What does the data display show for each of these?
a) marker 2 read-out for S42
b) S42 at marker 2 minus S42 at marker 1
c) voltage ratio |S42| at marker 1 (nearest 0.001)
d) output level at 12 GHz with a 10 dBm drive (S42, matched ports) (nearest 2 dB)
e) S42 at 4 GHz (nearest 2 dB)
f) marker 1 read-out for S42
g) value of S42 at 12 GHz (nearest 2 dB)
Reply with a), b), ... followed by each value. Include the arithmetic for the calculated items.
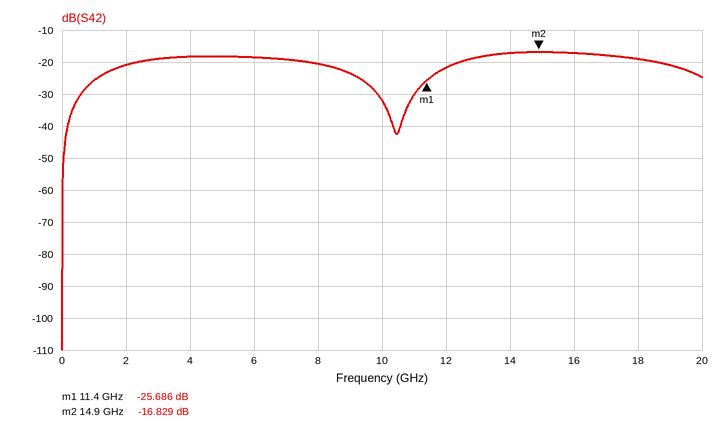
a) -16.829 dB
b) -16.829 − (-25.686) = 8.857 dB
c) 10^(-25.686/20) ≈ 0.052
d) 10 dBm + (-22 dB) = -12 dBm
e) -18 dB
f) -25.686 dB
g) -22 dB
